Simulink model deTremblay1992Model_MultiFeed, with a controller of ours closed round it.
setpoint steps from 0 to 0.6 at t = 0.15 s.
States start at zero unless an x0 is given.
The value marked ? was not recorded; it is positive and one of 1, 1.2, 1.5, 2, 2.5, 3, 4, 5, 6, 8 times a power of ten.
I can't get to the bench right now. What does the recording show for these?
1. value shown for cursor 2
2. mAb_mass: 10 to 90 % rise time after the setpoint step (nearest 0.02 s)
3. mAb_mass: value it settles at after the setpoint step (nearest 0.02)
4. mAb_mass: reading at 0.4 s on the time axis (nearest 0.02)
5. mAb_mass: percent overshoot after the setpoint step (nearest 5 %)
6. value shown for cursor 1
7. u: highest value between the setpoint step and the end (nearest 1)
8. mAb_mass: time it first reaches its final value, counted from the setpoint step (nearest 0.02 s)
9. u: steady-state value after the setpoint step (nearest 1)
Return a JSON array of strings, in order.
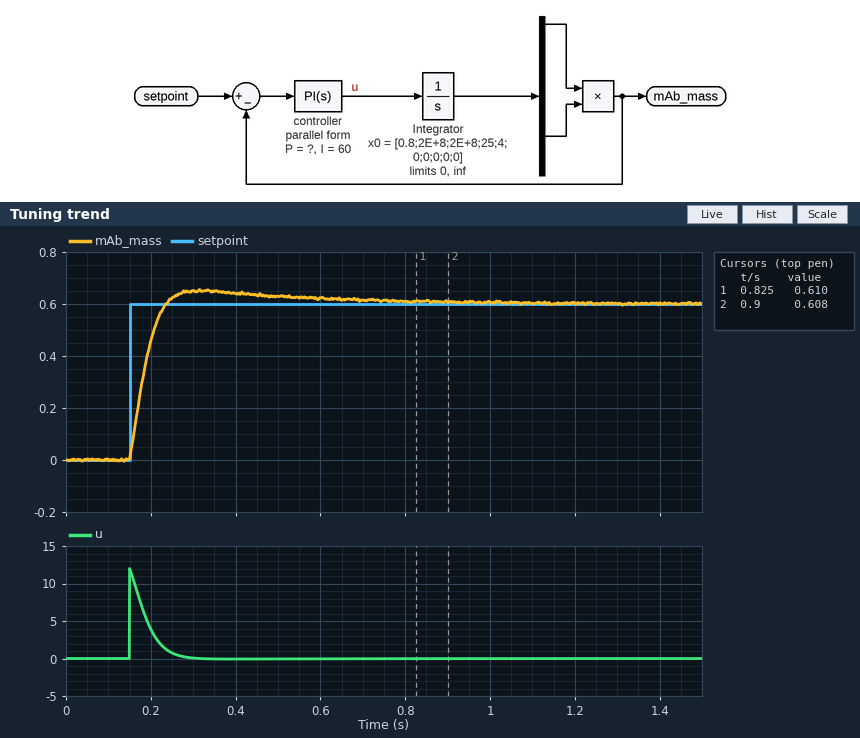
["0.608", "0.06 s", "0.60", "0.64", "10 %", "0.610", "12", "0.08 s", "0"]
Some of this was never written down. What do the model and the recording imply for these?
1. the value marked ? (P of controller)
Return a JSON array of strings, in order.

["20"]
